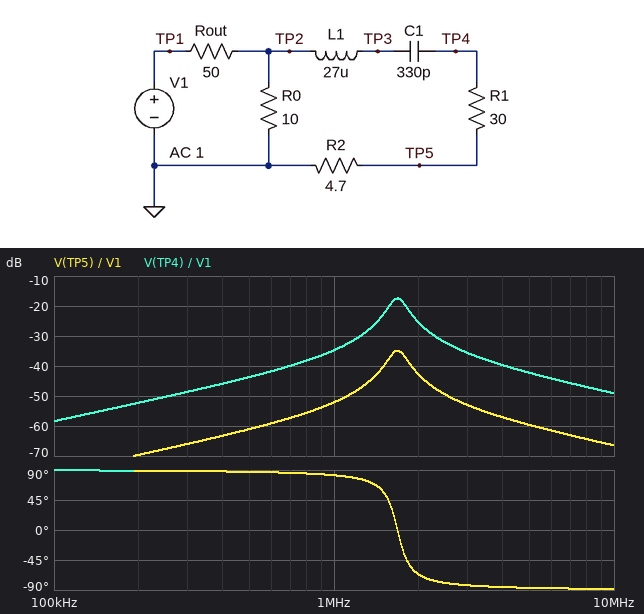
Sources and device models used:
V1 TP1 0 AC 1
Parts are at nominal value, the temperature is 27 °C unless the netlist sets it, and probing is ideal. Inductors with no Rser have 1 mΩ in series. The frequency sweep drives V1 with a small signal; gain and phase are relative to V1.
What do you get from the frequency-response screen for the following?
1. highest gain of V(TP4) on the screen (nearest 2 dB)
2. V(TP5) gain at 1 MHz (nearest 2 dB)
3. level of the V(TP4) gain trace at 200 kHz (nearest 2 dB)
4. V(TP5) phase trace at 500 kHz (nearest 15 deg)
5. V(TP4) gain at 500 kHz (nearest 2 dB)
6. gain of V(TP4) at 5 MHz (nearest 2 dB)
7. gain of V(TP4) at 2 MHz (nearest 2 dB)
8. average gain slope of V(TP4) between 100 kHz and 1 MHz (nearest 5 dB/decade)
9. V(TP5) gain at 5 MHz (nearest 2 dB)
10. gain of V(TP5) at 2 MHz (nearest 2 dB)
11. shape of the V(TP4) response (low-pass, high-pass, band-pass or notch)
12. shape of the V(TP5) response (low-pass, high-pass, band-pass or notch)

-18 dB
-52 dB
-52 dB
90 deg
-44 dB
-42 dB
-26 dB
25 dB/decade
-60 dB
-42 dB
band-pass
band-pass
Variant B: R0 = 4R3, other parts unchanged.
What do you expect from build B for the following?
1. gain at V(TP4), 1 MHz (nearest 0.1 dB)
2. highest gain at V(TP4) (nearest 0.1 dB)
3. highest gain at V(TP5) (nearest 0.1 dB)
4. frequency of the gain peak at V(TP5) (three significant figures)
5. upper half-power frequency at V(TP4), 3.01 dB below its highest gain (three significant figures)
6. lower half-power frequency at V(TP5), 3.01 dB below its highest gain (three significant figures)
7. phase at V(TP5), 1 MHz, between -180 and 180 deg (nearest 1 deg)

-41.2 dB
-23.0 dB
-40.3 dB
1.69 MHz
1.80 MHz
1.58 MHz
83 deg
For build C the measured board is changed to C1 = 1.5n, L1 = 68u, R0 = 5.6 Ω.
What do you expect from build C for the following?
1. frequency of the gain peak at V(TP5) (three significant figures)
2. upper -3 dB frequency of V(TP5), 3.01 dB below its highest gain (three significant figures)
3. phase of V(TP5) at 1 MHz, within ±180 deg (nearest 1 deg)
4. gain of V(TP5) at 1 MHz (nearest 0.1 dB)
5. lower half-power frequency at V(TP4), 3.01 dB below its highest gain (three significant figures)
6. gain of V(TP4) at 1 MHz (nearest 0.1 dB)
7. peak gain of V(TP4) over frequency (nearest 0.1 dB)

498 kHz
547 kHz
-83 deg
-56.7 dB
454 kHz
-39.3 dB
-21.1 dB
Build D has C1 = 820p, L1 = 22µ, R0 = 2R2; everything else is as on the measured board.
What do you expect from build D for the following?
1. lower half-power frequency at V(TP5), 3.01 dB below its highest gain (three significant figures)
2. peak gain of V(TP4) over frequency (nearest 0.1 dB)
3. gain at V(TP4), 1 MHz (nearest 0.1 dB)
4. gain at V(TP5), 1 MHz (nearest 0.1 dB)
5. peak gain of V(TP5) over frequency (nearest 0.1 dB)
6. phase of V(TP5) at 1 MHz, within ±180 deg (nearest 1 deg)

1.06 MHz
-28.0 dB
-33.2 dB
-50.6 dB
-45.4 dB
57 deg
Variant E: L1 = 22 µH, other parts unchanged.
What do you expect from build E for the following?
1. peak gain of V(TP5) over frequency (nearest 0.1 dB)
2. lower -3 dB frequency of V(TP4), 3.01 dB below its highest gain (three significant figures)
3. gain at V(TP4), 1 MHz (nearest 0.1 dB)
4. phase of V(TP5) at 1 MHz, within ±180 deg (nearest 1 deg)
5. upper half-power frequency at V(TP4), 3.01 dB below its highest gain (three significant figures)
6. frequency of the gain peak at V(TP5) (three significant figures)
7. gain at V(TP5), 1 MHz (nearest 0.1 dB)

-34.8 dB
1.72 MHz
-35.6 dB
83 deg
2.03 MHz
1.87 MHz
-52.9 dB
